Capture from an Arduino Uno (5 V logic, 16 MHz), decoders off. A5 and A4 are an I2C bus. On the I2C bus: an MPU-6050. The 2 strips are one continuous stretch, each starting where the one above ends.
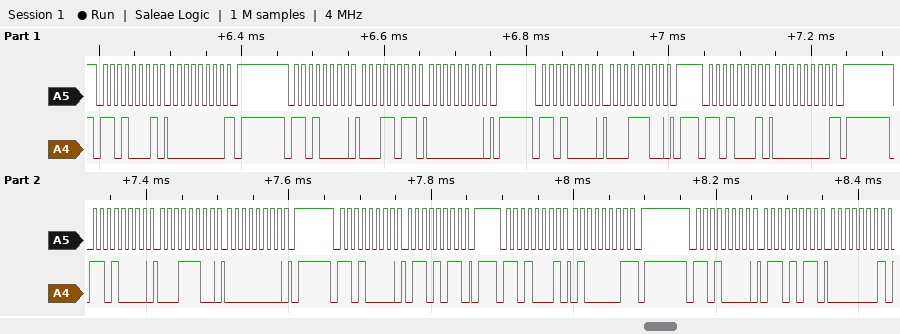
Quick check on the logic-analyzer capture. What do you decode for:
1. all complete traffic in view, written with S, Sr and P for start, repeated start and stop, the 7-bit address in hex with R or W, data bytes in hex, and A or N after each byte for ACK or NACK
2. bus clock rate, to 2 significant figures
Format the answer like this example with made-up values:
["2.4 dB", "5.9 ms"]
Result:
["S 68R A 00 N P S 68W A 1B A 00 A P S 68W A 1C A P S 68R A 00 N P S 68W A 1C A 00 A P S 68W A 6B A P S 68R A 41 N P S 68W A 6B A 01 A", "100 kHz"]
